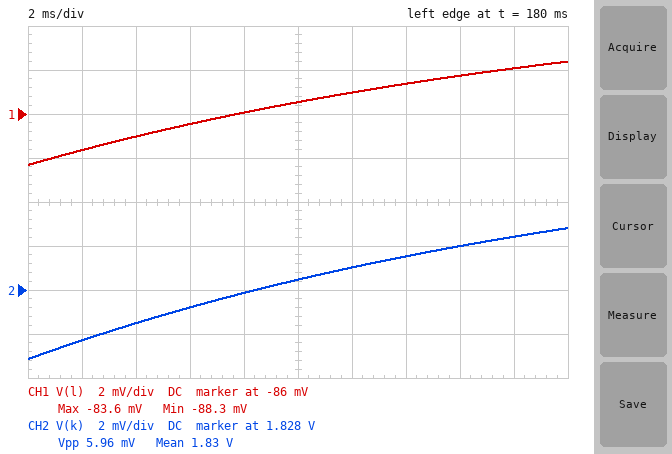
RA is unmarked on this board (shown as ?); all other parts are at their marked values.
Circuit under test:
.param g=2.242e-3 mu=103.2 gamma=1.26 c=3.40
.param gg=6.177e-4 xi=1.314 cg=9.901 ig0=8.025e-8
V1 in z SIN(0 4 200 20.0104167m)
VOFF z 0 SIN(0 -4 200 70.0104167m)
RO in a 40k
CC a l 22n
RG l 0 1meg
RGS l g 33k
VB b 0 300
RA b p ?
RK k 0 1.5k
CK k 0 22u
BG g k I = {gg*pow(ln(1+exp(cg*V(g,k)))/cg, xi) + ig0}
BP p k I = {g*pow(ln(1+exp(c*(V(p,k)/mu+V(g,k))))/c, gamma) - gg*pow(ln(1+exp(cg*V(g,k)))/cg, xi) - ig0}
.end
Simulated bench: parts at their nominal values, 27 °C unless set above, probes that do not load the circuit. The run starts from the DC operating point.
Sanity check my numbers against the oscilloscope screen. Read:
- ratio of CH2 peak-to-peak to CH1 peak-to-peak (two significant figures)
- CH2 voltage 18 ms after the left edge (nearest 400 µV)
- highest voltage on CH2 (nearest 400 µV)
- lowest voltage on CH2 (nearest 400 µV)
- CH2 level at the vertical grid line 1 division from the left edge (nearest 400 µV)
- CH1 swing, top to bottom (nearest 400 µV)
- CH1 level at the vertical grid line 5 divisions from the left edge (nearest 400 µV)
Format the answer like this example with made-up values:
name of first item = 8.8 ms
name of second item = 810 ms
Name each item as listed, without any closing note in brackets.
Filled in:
ratio of CH2 peak-to-peak to CH1 peak-to-peak = 1.3
CH2 voltage 18 ms after the left edge = 1.8304 V
highest voltage on CH2 = 1.8308 V
lowest voltage on CH2 = 1.8248 V
CH2 level at the vertical grid line 1 division from the left edge = 1.8256 V
CH1 swing, top to bottom = 4.8 mV
CH1 level at the vertical grid line 5 divisions from the left edge = -85.6 mV
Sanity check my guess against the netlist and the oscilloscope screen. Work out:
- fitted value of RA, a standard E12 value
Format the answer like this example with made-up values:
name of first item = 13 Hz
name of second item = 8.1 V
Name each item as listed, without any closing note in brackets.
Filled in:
fitted value of RA, a standard E12 value = 33 kΩ
